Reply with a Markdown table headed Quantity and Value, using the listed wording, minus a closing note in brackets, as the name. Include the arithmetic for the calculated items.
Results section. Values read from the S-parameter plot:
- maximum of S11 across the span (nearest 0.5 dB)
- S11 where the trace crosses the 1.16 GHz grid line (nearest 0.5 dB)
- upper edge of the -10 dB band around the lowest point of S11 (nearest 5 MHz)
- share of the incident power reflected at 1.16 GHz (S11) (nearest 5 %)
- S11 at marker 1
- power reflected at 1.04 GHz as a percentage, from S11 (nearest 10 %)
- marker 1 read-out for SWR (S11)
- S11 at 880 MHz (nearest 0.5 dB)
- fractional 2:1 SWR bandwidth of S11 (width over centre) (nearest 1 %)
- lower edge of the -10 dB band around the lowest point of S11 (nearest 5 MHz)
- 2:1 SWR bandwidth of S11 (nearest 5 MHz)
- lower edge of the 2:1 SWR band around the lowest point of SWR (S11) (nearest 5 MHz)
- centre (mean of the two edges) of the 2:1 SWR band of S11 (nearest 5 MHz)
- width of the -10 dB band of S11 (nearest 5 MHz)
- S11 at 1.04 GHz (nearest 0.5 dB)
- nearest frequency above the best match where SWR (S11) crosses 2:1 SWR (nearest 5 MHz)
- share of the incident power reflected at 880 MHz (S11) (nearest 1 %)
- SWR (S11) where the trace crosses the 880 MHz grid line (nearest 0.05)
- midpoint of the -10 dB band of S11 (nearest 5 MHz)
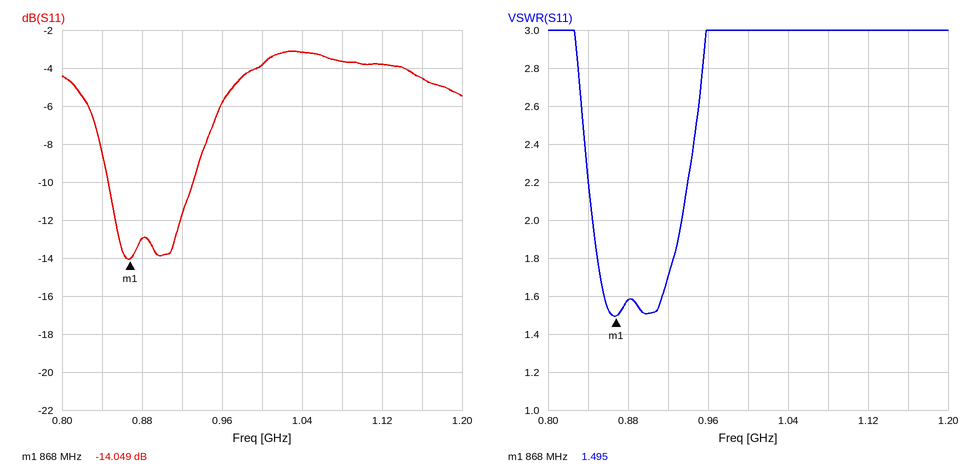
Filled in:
| Quantity | Value |
|---|---|
| maximum of S11 across the span | -3.0 dB |
| S11 where the trace crosses the 1.16 GHz grid line | -4.5 dB |
| upper edge of the -10 dB band around the lowest point of S11 | 930 MHz |
| share of the incident power reflected at 1.16 GHz (S11) | 10^(-4.5/10) ≈ 35 % |
| S11 at marker 1 | -14.049 dB |
| power reflected at 1.04 GHz as a percentage, from S11 | 10^(-3/10) ≈ 50 % |
| marker 1 read-out for SWR | 1.495 |
| S11 at 880 MHz | -13.0 dB |
| fractional 2:1 SWR bandwidth of S11 (width over centre) | 90 MHz / 890 MHz ≈ 10 % |
| lower edge of the -10 dB band around the lowest point of S11 | 845 MHz |
| 2:1 SWR bandwidth of S11 | 935 MHz − 845 MHz = 90 MHz |
| lower edge of the 2:1 SWR band around the lowest point of SWR (S11) | 845 MHz |
| centre (mean of the two edges) of the 2:1 SWR band of S11 | 890 MHz |
| width of the -10 dB band of S11 | 930 MHz − 845 MHz = 85 MHz |
| S11 at 1.04 GHz | -3.0 dB |
| nearest frequency above the best match where SWR (S11) crosses 2:1 SWR | 935 MHz |
| share of the incident power reflected at 880 MHz (S11) | 10^(-13/10) ≈ 5 % |
| SWR (S11) where the trace crosses the 880 MHz grid line | 1.60 |
| midpoint of the -10 dB band of S11 | 890 MHz |
